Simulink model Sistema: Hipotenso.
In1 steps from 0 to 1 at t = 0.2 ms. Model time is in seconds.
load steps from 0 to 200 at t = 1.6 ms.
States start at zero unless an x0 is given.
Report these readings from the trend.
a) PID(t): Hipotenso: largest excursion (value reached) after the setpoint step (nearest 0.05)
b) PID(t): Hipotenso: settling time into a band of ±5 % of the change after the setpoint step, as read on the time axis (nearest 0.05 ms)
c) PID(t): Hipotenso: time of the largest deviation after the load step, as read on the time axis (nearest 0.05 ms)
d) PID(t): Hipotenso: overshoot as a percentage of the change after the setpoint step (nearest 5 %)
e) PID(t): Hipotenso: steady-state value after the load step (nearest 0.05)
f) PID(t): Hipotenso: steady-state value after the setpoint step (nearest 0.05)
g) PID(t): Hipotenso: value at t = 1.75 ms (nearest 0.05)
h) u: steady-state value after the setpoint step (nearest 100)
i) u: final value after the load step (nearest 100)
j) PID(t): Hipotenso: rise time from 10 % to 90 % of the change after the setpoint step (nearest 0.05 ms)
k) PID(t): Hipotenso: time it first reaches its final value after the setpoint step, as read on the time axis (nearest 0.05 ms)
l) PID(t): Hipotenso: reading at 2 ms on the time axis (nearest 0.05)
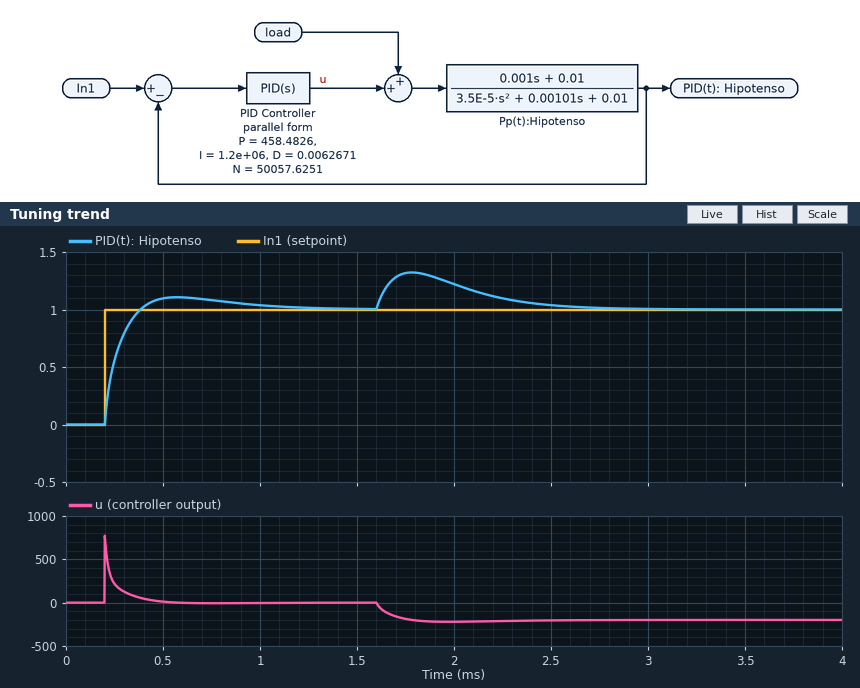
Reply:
1.10
0.90 ms
1.80 ms
10 %
1.00
1.00
1.30
0
-200
0.15 ms
0.40 ms
1.20
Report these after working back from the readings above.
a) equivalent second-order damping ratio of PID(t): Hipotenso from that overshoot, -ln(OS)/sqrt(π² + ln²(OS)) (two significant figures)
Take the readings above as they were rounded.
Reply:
0.59
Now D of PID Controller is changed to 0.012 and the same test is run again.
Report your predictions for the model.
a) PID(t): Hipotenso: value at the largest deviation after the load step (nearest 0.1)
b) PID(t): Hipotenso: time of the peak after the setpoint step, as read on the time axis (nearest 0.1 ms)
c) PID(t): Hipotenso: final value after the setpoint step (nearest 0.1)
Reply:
1.3
0.6 ms
1.0
